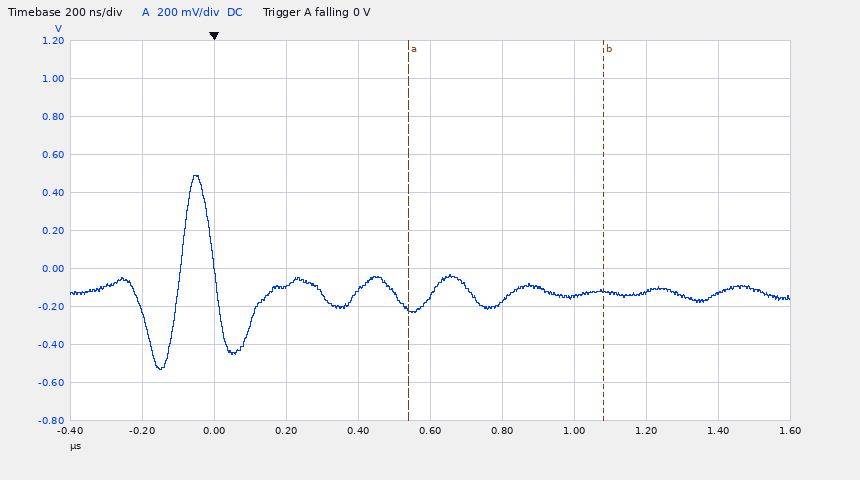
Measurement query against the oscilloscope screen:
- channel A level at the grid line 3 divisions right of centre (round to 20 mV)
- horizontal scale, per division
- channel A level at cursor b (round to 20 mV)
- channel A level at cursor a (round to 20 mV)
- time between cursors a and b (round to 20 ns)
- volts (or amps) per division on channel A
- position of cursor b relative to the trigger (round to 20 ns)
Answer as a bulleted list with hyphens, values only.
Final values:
- -120 mV
- 200 ns
- -120 mV
- -220 mV
- 540 ns
- 200 mV
- +1.08 µs
